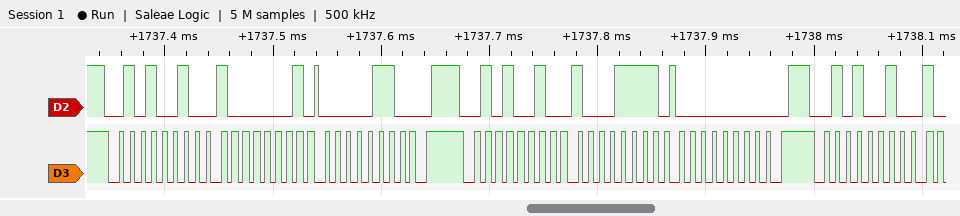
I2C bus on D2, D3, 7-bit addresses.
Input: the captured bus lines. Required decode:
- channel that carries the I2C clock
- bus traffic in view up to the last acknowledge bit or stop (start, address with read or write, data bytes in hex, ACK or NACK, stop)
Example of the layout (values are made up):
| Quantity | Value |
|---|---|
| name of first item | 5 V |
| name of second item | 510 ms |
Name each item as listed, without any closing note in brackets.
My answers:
| Quantity | Value |
|---|---|
| channel that carries the I2C clock | D3 |
| bus traffic in view up to the last acknowledge bit or stop | start, address 29 write ACK, 81 ACK, 06 ACK, stop, start, address 29 write ACK, 8F ACK, 00 ACK, stop, start, address 29 write ACK |
